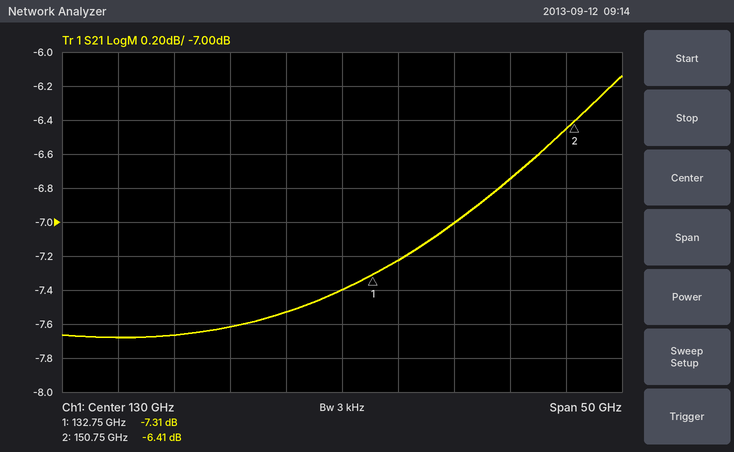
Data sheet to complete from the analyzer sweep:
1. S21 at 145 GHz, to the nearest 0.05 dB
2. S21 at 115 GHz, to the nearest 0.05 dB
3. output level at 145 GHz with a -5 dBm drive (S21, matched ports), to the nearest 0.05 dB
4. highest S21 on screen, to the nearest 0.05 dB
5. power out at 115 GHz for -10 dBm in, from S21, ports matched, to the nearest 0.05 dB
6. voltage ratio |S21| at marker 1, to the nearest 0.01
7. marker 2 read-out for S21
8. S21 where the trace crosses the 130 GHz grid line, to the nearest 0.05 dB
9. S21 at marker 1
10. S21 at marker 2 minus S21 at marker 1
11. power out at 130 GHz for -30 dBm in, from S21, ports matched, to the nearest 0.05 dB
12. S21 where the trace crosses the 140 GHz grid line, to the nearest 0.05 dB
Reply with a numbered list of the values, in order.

1. -6.75 dB
2. -7.65 dB
3. -11.75 dBm
4. -6.15 dB
5. -17.65 dBm
6. 0.43
7. -6.41 dB
8. -7.40 dB
9. -7.31 dB
10. 0.90 dB
11. -37.40 dBm
12. -7.00 dB
